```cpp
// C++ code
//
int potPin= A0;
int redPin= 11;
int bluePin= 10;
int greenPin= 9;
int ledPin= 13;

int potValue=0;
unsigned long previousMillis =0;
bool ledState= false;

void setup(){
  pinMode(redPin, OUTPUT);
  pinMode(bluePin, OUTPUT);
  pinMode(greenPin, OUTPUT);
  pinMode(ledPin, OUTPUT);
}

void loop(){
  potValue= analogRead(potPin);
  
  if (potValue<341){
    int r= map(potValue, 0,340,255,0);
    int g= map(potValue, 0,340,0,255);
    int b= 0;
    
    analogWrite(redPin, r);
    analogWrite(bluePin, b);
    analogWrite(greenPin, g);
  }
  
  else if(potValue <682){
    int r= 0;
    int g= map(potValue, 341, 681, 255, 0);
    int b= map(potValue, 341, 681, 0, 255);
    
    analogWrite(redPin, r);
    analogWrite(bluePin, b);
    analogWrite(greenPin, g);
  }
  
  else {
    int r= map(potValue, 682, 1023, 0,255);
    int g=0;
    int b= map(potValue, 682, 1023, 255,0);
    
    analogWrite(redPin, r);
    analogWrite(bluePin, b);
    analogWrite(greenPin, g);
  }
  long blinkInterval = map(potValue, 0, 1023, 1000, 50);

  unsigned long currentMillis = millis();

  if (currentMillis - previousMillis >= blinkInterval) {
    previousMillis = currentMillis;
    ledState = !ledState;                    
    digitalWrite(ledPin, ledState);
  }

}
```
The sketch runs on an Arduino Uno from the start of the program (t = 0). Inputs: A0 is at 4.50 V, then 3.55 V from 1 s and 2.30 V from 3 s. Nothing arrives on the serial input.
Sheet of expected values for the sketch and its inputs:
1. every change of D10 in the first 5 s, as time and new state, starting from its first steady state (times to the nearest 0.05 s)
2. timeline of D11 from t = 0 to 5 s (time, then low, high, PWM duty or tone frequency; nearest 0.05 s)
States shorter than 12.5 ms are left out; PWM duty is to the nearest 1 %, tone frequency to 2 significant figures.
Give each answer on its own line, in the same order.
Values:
0 s PWM 30 %; 1 s PWM 87 %; 3 s PWM 38 %
0 s PWM 70 %; 1 s PWM 13 %; 3 s low
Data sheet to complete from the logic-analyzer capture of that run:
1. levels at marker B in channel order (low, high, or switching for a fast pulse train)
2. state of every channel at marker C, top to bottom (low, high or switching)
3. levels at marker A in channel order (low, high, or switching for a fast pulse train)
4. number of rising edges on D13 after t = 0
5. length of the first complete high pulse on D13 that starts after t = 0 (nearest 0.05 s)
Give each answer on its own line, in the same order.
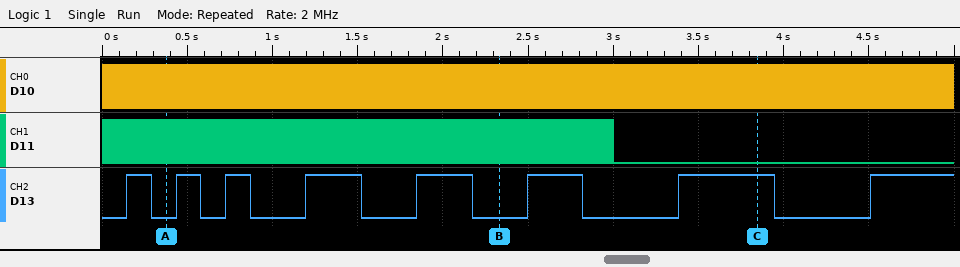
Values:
D10 switching, D11 switching, D13 low
D10 switching, D11 low, D13 high
D10 switching, D11 switching, D13 low
8
0.15 s
